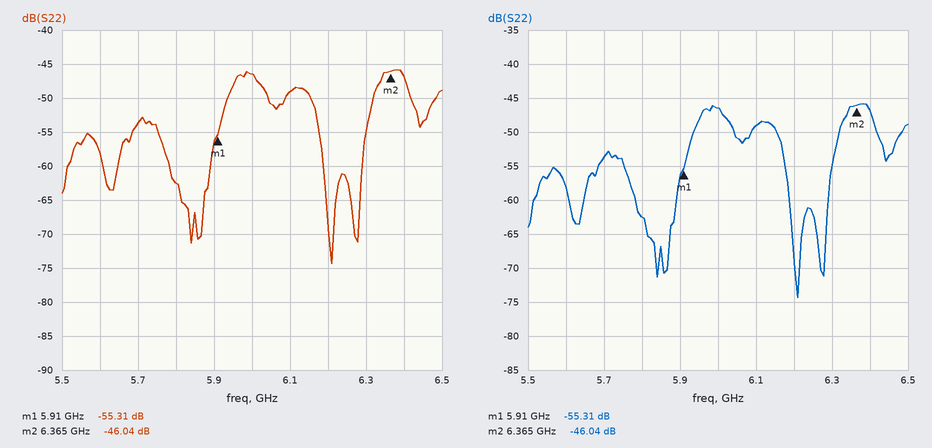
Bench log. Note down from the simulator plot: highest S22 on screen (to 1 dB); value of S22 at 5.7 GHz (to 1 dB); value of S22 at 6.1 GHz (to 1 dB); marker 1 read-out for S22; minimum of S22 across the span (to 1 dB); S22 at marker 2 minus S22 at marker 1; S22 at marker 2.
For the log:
-46 dB
-54 dB
-49 dB
-55.31 dB
-74 dB
9.27 dB
-46.04 dB
